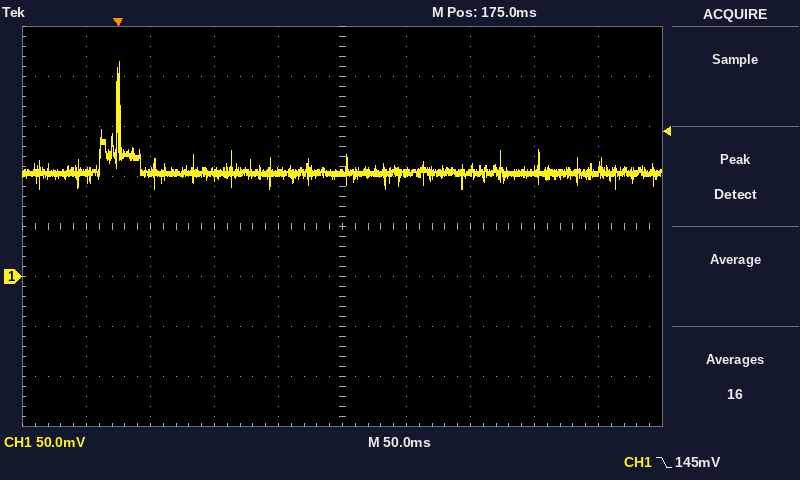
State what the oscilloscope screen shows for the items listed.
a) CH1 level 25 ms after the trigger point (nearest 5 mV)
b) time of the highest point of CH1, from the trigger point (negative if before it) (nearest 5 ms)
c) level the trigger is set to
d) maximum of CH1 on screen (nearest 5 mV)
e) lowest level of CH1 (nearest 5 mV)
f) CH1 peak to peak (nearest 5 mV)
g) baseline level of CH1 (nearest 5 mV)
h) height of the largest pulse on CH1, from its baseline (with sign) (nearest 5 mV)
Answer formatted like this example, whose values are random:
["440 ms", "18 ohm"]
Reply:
["105 mV", "0 ms", "145 mV", "215 mV", "90 mV", "125 mV", "105 mV", "+110 mV"]
